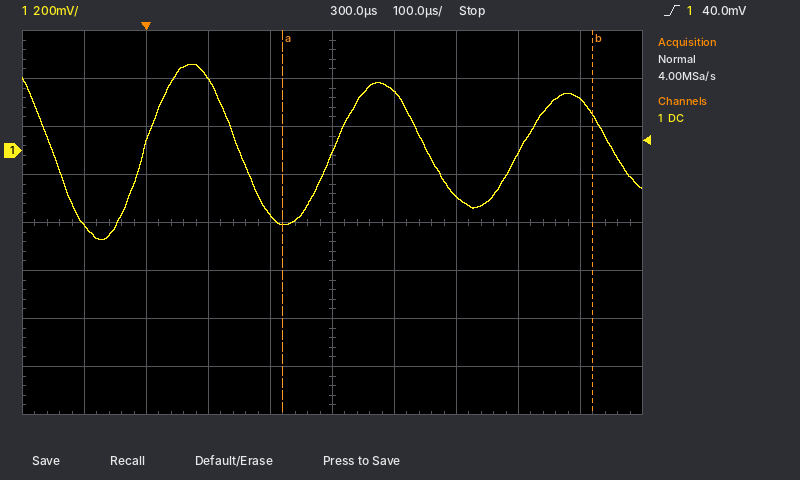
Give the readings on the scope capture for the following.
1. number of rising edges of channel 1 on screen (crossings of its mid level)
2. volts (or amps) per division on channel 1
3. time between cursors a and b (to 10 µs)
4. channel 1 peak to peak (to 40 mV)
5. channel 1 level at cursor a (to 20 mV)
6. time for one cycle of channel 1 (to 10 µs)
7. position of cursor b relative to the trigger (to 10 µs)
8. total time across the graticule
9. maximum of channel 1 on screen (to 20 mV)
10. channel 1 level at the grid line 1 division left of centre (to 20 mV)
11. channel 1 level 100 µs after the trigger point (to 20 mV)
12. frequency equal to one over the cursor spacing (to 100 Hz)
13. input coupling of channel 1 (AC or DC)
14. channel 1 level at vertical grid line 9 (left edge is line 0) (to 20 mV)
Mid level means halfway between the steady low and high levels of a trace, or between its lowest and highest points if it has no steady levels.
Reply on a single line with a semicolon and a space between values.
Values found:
3; 200 mV; 500 µs; 720 mV; -300 mV; 300 µs; +720 µs; 1 ms; 360 mV; -260 mV; 300 mV; 2.0 kHz; DC; 220 mV
